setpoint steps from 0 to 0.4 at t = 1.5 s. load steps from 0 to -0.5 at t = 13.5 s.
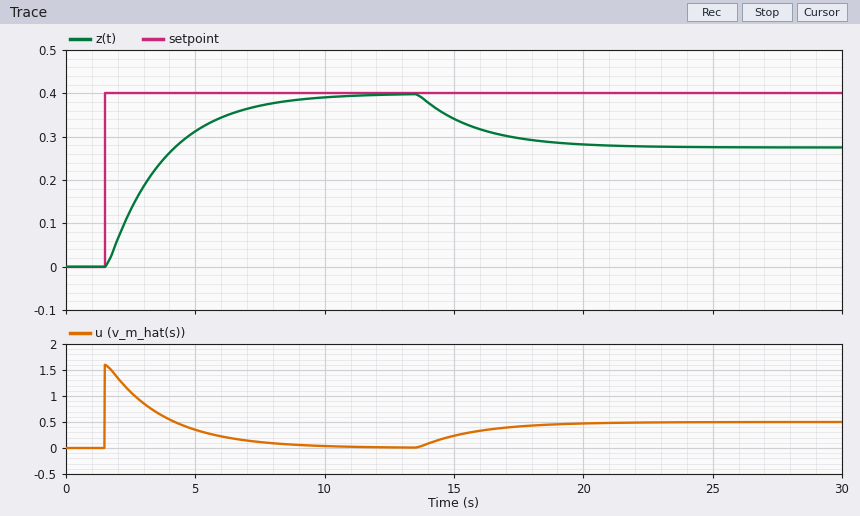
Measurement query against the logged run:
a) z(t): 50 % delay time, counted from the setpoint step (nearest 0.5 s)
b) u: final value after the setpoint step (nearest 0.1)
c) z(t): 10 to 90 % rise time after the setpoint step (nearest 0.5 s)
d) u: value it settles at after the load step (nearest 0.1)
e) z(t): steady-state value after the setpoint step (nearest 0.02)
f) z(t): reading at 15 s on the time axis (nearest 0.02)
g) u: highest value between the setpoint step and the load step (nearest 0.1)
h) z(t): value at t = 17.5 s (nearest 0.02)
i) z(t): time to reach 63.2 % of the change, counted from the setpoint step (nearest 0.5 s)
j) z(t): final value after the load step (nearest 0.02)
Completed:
1.5 s
0.0
5.0 s
0.5
0.40
0.34
1.6
0.30
2.5 s
0.28
